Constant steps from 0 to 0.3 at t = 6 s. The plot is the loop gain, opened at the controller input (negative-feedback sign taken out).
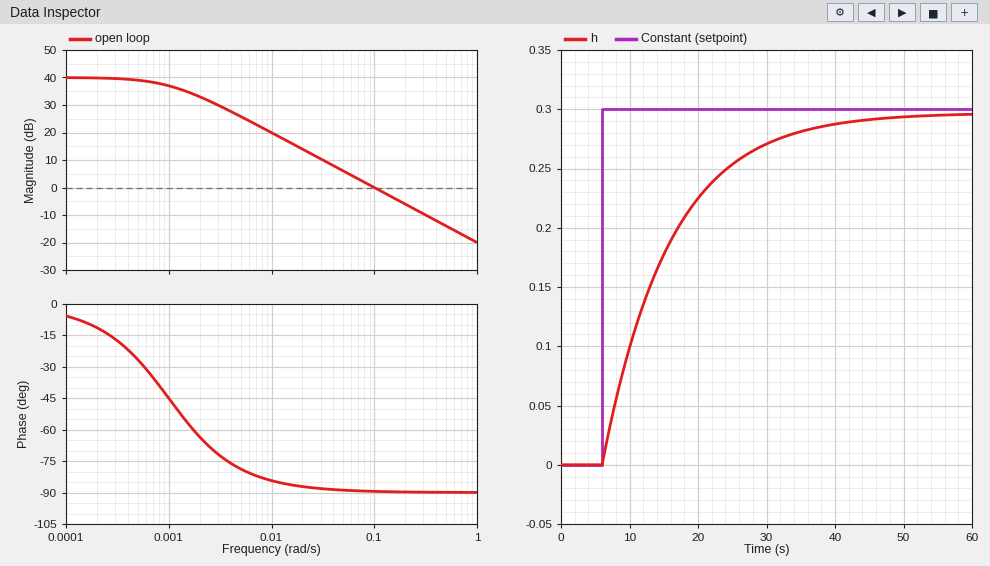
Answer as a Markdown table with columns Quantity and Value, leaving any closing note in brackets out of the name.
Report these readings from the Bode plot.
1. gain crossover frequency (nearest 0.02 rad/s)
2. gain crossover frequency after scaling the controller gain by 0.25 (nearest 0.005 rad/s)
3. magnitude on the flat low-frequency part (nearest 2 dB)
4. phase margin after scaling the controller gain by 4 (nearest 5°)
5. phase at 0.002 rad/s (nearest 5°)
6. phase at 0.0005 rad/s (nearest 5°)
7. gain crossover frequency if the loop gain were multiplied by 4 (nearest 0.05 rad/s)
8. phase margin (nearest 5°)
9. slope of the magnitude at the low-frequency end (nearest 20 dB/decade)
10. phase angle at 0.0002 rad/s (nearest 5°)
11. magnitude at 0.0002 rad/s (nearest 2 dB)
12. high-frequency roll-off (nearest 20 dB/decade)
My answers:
| Quantity | Value |
|---|---|
| gain crossover frequency | 0.10 rad/s |
| gain crossover frequency after scaling the controller gain by 0.25 | 0.025 rad/s |
| magnitude on the flat low-frequency part | 40 dB |
| phase margin after scaling the controller gain by 4 | 90° |
| phase at 0.002 rad/s | -65° |
| phase at 0.0005 rad/s | -25° |
| gain crossover frequency if the loop gain were multiplied by 4 | 0.40 rad/s |
| phase margin | 90° |
| slope of the magnitude at the low-frequency end | 0 dB/decade |
| phase angle at 0.0002 rad/s | -10° |
| magnitude at 0.0002 rad/s | 40 dB |
| high-frequency roll-off | -20 dB/decade |
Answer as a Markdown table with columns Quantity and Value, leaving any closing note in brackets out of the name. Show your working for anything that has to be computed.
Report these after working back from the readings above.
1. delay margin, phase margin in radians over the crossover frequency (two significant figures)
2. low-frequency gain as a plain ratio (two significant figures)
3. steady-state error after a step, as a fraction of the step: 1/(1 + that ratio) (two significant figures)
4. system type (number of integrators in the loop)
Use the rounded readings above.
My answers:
| Quantity | Value |
|---|---|
| delay margin, phase margin in radians over the crossover frequency | 90 × π / 180 / 0.1 = 16 s |
| low-frequency gain as a plain ratio | 10^(40 / 20) = 100 |
| steady-state error after a step, as a fraction of the step: 1/(1 + that ratio) | 1 / (1 + 100) = 0.0099 |
| system type | 0 |
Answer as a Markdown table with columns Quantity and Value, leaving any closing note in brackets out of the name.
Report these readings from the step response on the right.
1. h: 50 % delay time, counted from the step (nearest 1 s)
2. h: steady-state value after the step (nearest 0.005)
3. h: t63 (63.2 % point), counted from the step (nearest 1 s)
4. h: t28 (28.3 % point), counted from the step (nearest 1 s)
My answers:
| Quantity | Value |
|---|---|
| h: 50 % delay time, counted from the step | 7 s |
| h: steady-state value after the step | 0.295 |
| h: t63 (63.2 % point), counted from the step | 10 s |
| h: t28 (28.3 % point), counted from the step | 3 s |
